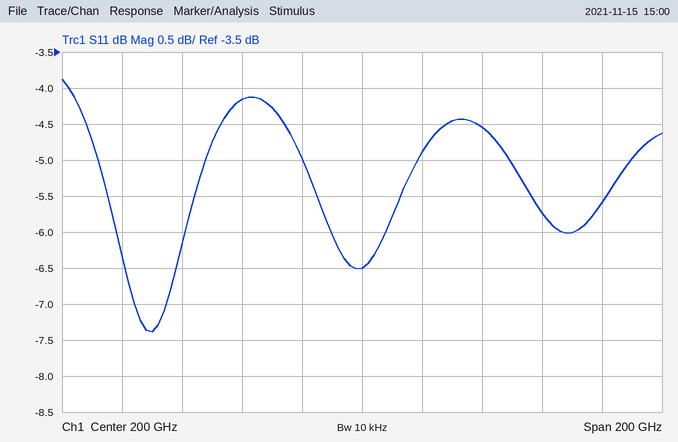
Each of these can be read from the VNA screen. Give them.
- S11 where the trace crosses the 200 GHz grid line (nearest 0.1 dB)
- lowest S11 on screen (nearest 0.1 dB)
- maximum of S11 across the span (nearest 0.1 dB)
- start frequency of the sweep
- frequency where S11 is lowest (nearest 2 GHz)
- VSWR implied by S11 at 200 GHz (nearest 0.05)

-6.5 dB
-7.4 dB
-3.9 dB
100 GHz
130 GHz
2.80
